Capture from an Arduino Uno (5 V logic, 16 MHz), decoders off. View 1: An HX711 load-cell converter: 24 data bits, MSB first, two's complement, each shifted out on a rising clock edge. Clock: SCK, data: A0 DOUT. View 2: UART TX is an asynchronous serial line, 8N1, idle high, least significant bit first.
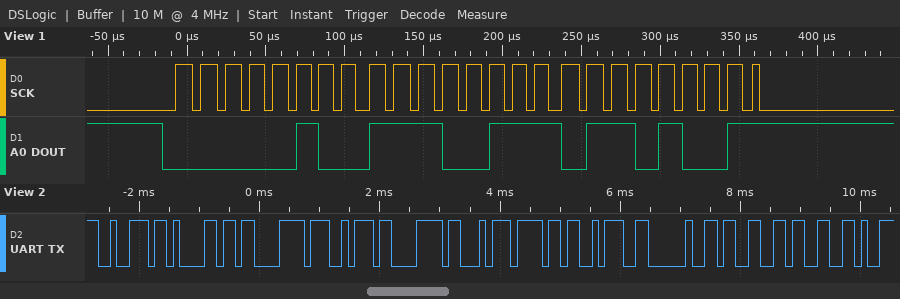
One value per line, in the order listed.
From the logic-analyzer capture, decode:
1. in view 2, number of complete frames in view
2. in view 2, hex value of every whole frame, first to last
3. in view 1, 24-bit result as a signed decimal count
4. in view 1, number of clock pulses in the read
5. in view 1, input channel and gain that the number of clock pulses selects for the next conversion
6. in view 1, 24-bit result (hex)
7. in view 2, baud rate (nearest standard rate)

11
0x72 0x61 0xC3 0xA7 0xC3 0xA3 0x6F 0x3A 0x20 0x33 0x33
321385
25
channel A, gain 128
0x04E769
9600 baud
